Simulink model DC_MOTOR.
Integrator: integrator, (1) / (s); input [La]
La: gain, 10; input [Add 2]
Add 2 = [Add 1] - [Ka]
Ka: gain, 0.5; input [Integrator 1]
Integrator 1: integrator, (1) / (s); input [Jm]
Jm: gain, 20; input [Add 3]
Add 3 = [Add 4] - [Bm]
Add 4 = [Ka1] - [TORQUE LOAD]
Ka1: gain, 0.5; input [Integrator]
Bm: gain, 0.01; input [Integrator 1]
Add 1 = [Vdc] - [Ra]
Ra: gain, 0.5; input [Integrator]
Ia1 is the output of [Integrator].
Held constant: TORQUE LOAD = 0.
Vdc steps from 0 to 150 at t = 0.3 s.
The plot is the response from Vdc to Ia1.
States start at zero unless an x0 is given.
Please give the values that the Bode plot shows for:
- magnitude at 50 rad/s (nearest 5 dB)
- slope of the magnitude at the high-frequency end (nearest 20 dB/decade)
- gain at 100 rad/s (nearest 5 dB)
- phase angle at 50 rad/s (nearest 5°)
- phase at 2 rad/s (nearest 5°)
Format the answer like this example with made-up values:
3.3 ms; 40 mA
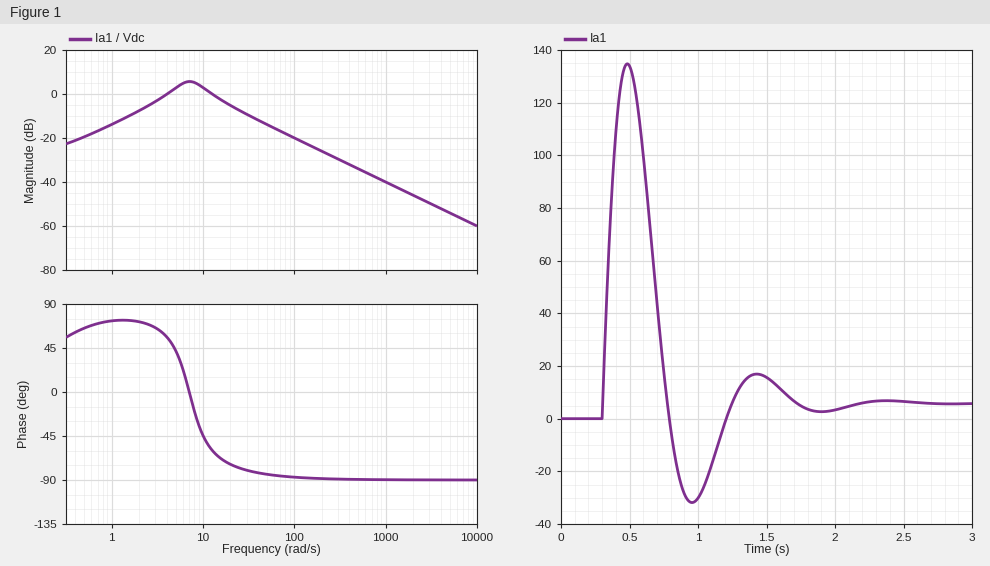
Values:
-15 dB; -20 dB/decade; -20 dB; -85°; 70°
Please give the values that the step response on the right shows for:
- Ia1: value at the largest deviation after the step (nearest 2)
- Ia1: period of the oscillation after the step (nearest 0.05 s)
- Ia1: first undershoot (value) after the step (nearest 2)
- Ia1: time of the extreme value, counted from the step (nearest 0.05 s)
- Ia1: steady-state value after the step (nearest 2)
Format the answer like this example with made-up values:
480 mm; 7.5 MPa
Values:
134; 0.95 s; -32; 0.20 s; 6
